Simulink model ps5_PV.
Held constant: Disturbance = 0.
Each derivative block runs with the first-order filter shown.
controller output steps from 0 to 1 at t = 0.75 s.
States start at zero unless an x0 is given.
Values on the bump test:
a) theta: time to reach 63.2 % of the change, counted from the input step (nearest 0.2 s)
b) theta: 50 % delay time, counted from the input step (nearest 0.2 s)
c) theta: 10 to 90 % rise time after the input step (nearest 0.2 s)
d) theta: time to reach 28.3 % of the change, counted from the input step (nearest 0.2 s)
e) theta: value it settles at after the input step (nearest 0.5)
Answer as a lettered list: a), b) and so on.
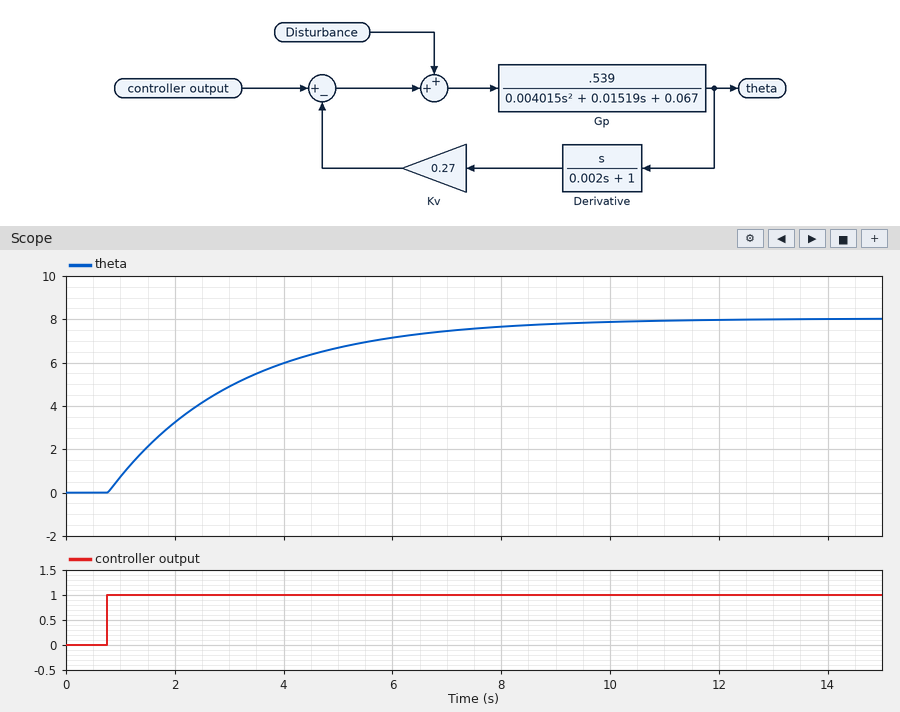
a) 2.4 s
b) 1.6 s
c) 5.2 s
d) 0.8 s
e) 8.0
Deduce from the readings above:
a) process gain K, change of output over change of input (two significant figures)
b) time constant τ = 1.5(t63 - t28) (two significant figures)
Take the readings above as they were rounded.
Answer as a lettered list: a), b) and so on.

a) 8.0
b) 2.4 s
